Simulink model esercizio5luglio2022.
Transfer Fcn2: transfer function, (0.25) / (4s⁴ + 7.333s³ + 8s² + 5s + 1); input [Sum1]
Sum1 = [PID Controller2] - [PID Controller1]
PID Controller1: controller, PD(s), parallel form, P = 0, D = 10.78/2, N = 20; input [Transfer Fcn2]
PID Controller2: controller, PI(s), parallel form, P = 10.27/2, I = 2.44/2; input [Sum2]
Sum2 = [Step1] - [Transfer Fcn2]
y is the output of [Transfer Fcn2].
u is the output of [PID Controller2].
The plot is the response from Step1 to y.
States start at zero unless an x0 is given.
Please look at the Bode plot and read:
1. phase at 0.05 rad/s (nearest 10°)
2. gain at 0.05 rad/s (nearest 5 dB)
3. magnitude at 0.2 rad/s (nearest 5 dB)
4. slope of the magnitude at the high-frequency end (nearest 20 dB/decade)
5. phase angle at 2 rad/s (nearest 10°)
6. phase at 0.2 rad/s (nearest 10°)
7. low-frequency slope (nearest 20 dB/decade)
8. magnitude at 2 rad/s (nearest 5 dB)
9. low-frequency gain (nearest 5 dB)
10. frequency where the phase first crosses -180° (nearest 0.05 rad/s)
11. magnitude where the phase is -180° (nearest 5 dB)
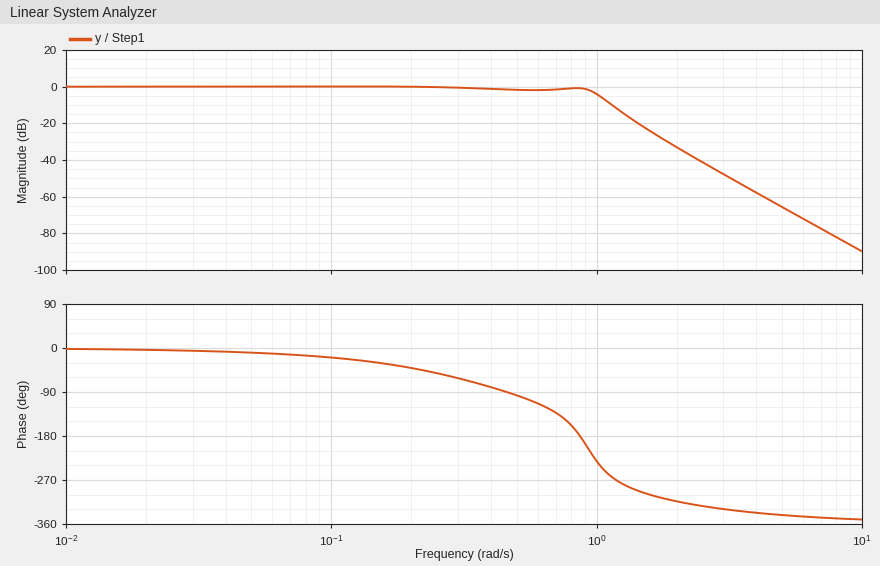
-10°
0 dB
0 dB
-80 dB/decade
-310°
-40°
0 dB/decade
-35 dB
0 dB
0.85 rad/s
0 dB
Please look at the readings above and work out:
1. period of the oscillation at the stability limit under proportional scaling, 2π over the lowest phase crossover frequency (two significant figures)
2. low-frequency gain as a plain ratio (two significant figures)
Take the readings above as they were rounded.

7.4 s
1.0
